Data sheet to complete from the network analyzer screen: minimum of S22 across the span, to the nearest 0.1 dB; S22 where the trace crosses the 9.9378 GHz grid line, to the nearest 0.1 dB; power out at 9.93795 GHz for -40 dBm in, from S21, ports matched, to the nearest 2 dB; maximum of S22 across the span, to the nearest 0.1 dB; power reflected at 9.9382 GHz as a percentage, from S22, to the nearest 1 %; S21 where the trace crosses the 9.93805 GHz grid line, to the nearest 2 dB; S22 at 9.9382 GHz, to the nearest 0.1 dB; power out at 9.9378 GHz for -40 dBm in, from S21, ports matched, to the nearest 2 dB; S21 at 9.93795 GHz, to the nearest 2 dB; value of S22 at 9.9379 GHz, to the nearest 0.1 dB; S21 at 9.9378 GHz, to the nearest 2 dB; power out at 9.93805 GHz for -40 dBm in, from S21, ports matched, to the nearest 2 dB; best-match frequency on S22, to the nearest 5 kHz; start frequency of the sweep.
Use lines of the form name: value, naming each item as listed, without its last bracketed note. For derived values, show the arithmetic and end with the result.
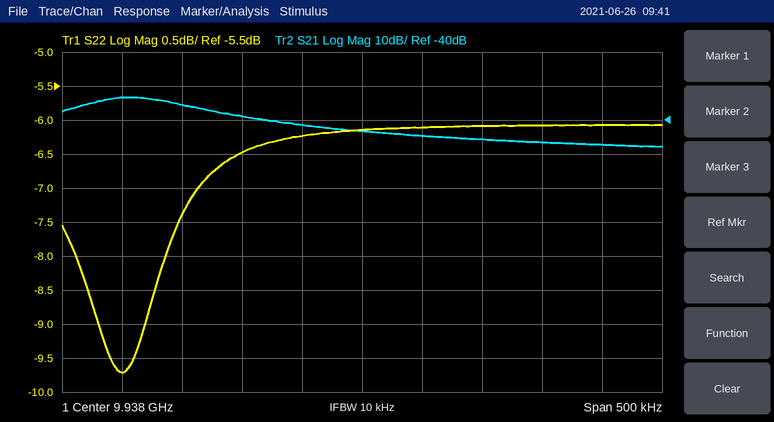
minimum of S22 across the span, to the nearest 0.1 dB: -9.7 dB
S22 where the trace crosses the 9.9378 GHz grid line, to the nearest 0.1 dB: -9.7 dB
power out at 9.93795 GHz for -40 dBm in, from S21, ports matched, to the nearest 2 dB: -40 dBm + (-42 dB) = -82 dBm
maximum of S22 across the span, to the nearest 0.1 dB: -6.1 dB
power reflected at 9.9382 GHz as a percentage, from S22, to the nearest 1 %: 10^(-6.1/10) ≈ 25 %
S21 where the trace crosses the 9.93805 GHz grid line, to the nearest 2 dB: -44 dB
S22 at 9.9382 GHz, to the nearest 0.1 dB: -6.1 dB
power out at 9.9378 GHz for -40 dBm in, from S21, ports matched, to the nearest 2 dB: -40 dBm + (-34 dB) = -74 dBm
S21 at 9.93795 GHz, to the nearest 2 dB: -42 dB
value of S22 at 9.9379 GHz, to the nearest 0.1 dB: -6.5 dB
S21 at 9.9378 GHz, to the nearest 2 dB: -34 dB
power out at 9.93805 GHz for -40 dBm in, from S21, ports matched, to the nearest 2 dB: -40 dBm + (-44 dB) = -84 dBm
best-match frequency on S22, to the nearest 5 kHz: 9.937800 GHz
start frequency of the sweep: 9.93775 GHz
